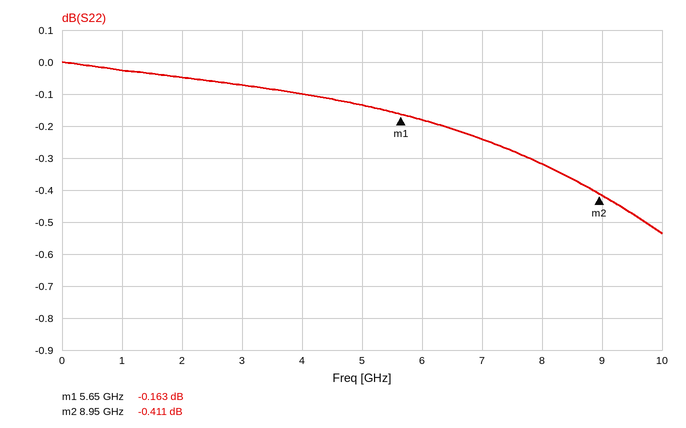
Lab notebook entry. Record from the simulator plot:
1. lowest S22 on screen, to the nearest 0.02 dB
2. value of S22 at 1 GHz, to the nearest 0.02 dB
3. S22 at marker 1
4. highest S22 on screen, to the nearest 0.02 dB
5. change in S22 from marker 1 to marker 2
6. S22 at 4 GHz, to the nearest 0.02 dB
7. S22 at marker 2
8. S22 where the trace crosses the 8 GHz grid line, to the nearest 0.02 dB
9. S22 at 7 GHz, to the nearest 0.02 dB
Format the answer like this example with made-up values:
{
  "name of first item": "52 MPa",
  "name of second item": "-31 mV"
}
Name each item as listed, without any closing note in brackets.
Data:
{
  "lowest S22 on screen, to the nearest 0.02 dB": "-0.54 dB",
  "value of S22 at 1 GHz, to the nearest 0.02 dB": "-0.02 dB",
  "S22 at marker 1": "-0.163 dB",
  "highest S22 on screen, to the nearest 0.02 dB": "0.00 dB",
  "change in S22 from marker 1 to marker 2": "-0.248 dB",
  "S22 at 4 GHz, to the nearest 0.02 dB": "-0.10 dB",
  "S22 at marker 2": "-0.411 dB",
  "S22 where the trace crosses the 8 GHz grid line, to the nearest 0.02 dB": "-0.32 dB",
  "S22 at 7 GHz, to the nearest 0.02 dB": "-0.24 dB"
}
